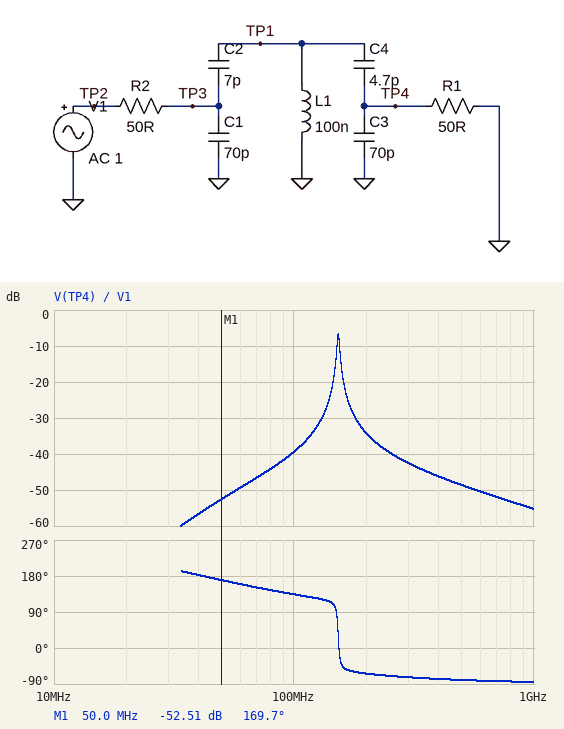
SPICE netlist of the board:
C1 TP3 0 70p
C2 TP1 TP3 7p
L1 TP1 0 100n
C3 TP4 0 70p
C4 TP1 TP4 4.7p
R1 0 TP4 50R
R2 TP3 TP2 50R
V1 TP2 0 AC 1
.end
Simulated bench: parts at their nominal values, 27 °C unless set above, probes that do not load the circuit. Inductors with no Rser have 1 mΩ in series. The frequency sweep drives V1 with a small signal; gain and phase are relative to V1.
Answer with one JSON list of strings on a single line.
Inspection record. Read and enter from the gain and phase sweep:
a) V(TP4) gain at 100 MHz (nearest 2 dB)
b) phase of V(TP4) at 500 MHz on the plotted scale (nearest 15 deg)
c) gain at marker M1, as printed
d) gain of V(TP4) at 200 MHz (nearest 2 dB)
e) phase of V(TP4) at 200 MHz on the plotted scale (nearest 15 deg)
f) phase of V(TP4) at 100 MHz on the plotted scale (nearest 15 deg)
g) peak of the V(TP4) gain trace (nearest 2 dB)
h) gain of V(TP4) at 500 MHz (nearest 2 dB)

["-40 dB", "-75 deg", "-52.51 dB", "-34 dB", "-60 deg", "135 deg", "-6 dB", "-48 dB"]
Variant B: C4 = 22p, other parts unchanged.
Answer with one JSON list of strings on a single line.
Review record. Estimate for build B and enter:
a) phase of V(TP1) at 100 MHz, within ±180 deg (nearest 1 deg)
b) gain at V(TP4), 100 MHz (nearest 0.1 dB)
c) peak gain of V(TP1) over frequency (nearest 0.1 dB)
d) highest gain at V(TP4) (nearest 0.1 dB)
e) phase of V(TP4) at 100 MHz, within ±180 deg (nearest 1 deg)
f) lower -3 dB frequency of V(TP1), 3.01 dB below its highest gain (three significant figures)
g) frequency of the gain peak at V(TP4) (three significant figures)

["63 deg", "-12.1 dB", "3.2 dB", "-9.7 dB", "82 deg", "99.4 MHz", "103 MHz"]
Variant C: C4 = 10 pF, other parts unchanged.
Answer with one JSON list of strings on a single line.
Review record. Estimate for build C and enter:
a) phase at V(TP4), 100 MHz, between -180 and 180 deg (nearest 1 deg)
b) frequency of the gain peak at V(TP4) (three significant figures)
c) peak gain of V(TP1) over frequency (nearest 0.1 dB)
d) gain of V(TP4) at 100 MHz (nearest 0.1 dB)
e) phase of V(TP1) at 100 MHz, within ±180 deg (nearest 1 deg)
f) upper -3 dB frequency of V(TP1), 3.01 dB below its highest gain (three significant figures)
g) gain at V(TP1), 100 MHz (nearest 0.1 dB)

["130 deg", "129 MHz", "12.0 dB", "-30.1 dB", "109 deg", "131 MHz", "-11.4 dB"]
